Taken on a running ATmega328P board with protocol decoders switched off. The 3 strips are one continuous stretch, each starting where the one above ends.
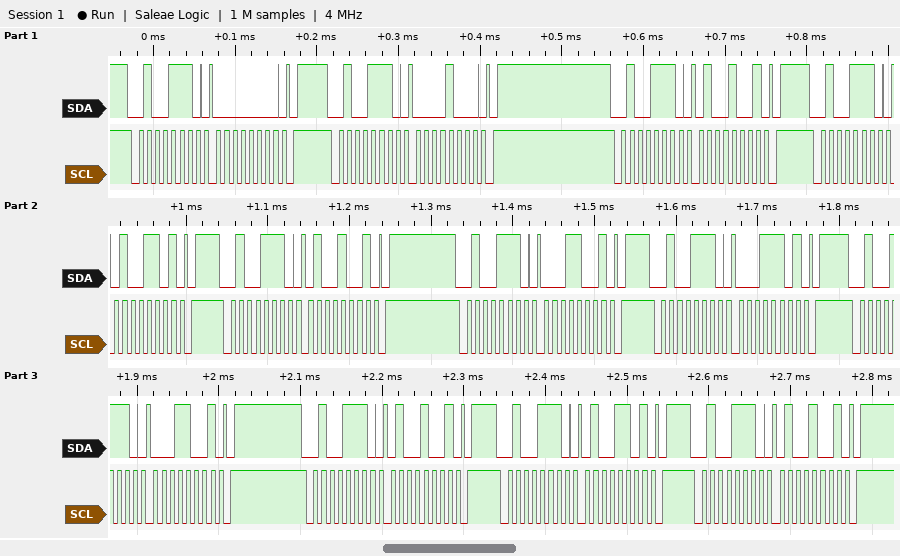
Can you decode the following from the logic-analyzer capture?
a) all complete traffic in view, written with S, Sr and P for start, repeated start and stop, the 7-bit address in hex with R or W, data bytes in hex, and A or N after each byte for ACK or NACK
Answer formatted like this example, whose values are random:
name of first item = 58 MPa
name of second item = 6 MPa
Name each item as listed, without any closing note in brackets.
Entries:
all complete traffic in view, written with S, Sr and P for start, repeated start and stop, the 7-bit address in hex with R or W, data bytes in hex, and A or N after each byte for ACK or NACK = S 27W A 00 A P S 27W A 08 A P S 27W A 49 A P S 27W A 4D A P S 27W A 49 A P S 27W A 19 A P S 27W A 1D A P S 27W A 19 A P S 27W A 49 A P S 27W A 4D A P S 27W A 49 A P
